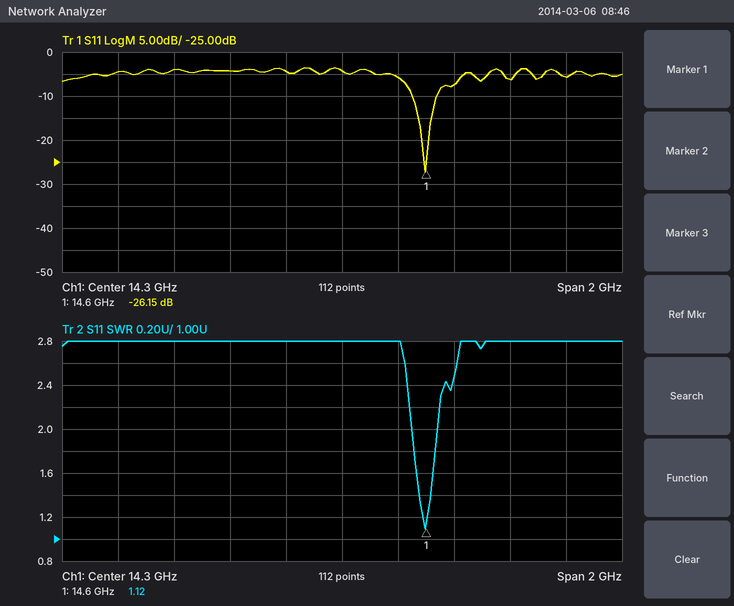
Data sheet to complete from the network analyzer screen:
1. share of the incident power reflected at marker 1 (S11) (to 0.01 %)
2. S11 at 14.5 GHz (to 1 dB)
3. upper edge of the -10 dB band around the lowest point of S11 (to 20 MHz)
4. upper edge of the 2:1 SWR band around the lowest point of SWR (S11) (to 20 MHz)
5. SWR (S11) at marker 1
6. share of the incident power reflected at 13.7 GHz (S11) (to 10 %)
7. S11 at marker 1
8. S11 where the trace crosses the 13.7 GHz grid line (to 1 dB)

0.24 %
-6 dB
14.64 GHz
14.64 GHz
1.12
40 %
-26.15 dB
-4 dB
